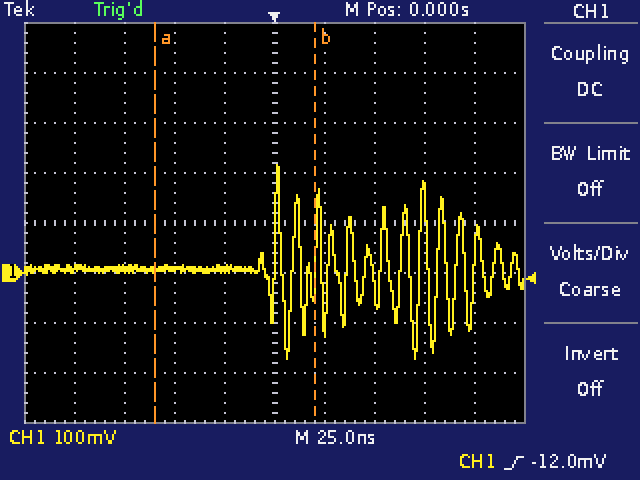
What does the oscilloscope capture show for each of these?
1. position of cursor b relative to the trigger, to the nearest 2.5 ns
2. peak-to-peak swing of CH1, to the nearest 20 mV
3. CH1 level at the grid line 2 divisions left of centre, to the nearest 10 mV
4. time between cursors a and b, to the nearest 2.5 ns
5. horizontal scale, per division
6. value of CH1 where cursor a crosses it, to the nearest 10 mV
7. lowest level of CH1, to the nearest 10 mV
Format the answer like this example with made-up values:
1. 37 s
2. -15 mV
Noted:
1. +20.0 ns
2. 380 mV
3. 10 mV
4. 80.0 ns
5. 25 ns
6. 10 mV
7. -170 mV
